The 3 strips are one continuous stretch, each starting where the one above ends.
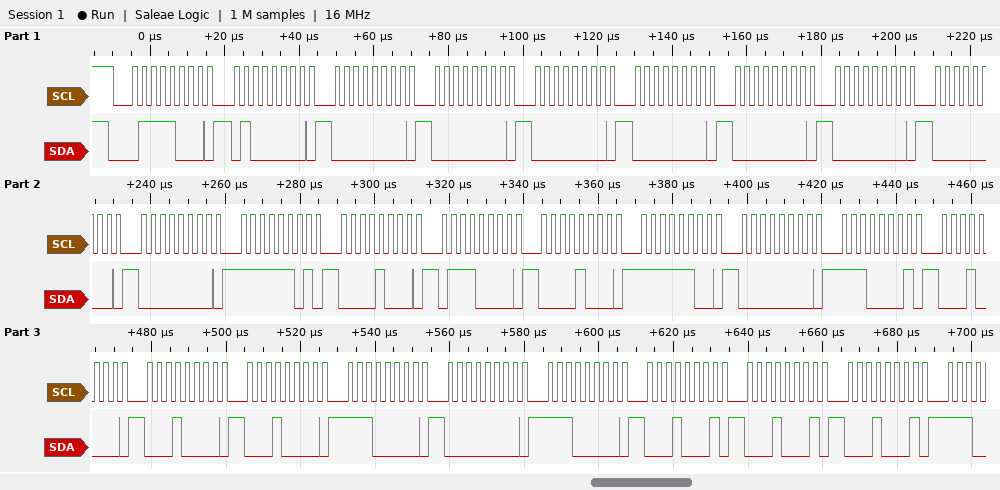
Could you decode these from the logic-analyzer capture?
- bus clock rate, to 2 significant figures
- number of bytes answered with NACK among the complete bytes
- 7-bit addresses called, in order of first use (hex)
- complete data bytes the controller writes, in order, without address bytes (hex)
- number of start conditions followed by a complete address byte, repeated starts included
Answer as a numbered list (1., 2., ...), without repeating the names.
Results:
1. 400 kHz
2. 0
3. 0x3C
4. 40 00 00 00 00 00 00 00 00 FD 08 70 08 FC 00 E1 10 10 10 E0 00 E0 11 11 11
5. 1
